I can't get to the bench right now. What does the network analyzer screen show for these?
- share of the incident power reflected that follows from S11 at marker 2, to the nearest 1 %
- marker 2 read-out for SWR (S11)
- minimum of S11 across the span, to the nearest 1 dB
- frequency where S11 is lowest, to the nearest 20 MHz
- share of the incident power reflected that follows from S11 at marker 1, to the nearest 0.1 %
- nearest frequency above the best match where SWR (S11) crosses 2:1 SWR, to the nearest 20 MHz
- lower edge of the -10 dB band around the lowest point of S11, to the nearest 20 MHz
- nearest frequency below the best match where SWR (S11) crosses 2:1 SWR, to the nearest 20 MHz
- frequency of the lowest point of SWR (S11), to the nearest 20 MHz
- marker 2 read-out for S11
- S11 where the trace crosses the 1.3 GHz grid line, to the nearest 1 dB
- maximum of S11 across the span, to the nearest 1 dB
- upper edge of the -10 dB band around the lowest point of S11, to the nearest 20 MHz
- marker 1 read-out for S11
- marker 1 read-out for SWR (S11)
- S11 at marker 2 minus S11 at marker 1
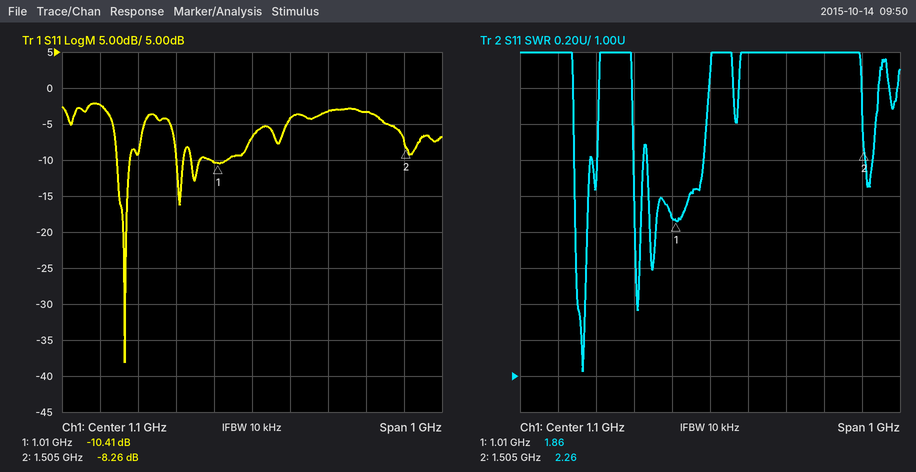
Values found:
15 %
2.26
-38 dB
760 MHz
9.1 %
780 MHz
740 MHz
740 MHz
760 MHz
-8.26 dB
-3 dB
-2 dB
780 MHz
-10.41 dB
1.86
2.15 dB
